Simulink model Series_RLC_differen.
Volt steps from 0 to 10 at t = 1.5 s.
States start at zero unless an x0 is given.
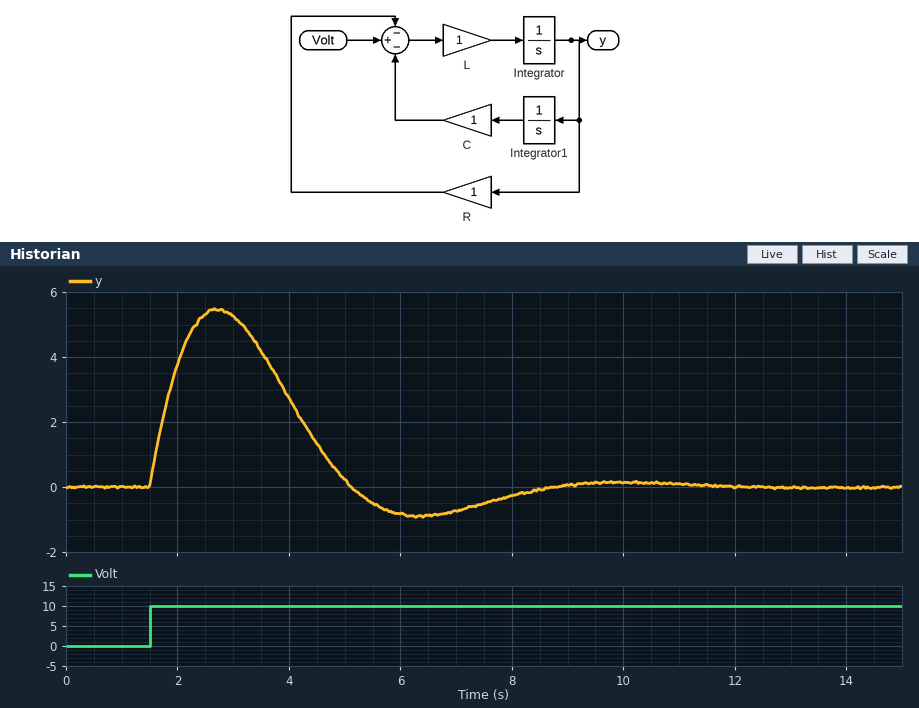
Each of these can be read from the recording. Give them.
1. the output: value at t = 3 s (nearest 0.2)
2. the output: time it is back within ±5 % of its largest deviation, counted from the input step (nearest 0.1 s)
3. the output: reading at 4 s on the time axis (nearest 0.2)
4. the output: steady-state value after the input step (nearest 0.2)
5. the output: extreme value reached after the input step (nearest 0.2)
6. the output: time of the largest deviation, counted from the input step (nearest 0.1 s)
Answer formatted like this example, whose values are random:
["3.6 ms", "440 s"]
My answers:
["5.2", "6.5 s", "2.8", "0.0", "5.4", "1.2 s"]
